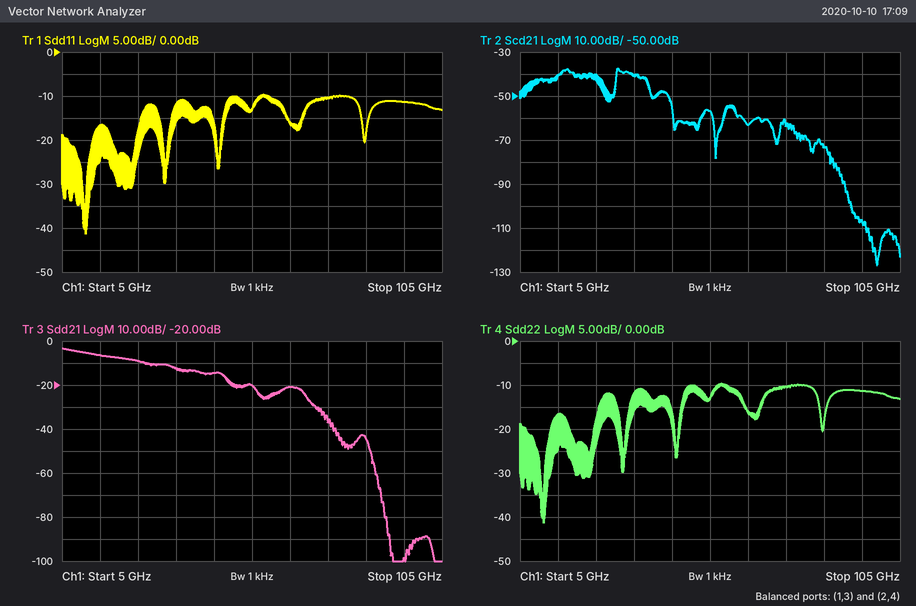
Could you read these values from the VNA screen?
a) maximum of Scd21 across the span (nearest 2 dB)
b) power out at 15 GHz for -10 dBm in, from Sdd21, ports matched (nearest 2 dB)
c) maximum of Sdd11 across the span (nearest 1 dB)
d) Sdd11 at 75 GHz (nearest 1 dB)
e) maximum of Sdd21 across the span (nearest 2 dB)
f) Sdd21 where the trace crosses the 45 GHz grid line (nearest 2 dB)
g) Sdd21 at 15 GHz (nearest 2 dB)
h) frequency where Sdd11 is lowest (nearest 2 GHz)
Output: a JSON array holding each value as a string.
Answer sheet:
["-38 dB", "-16 dBm", "-10 dB", "-10 dB", "-4 dB", "-14 dB", "-6 dB", "12 GHz"]
